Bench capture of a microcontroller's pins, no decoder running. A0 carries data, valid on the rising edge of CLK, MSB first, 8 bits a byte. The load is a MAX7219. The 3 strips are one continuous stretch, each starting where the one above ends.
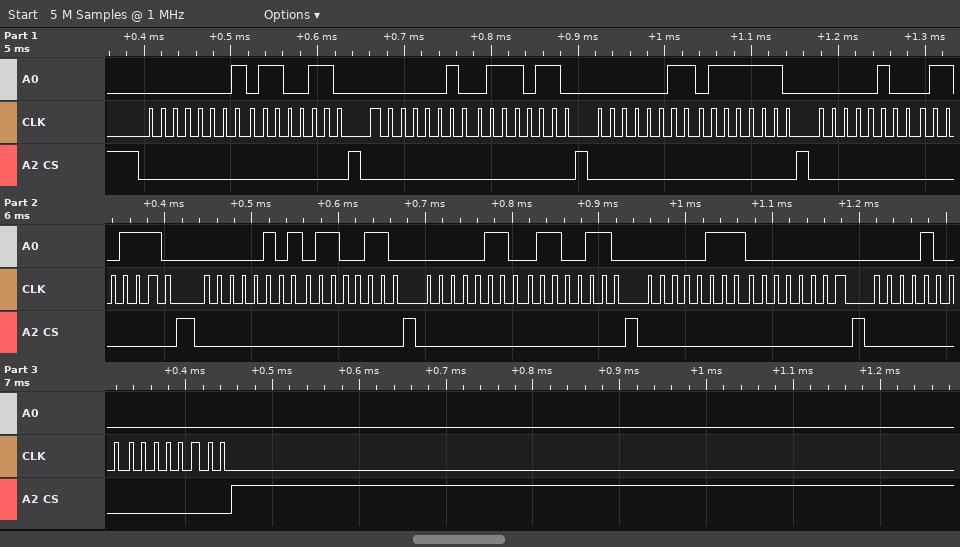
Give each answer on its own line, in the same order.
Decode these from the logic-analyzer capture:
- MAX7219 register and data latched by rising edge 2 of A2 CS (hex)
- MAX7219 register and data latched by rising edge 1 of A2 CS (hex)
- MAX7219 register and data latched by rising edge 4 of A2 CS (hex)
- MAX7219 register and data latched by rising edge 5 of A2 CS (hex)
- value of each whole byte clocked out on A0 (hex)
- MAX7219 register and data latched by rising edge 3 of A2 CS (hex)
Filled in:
register 0x2, data 0x76
register 0x1, data 0x66
register 0x4, data 0x6E
register 0x5, data 0x66
0x01 0x66 0x02 0x76 0x03 0x7E 0x04 0x6E 0x05 0x66 0x06 0x66 0x07 0x00 0x08 0x00
register 0x3, data 0x7E
